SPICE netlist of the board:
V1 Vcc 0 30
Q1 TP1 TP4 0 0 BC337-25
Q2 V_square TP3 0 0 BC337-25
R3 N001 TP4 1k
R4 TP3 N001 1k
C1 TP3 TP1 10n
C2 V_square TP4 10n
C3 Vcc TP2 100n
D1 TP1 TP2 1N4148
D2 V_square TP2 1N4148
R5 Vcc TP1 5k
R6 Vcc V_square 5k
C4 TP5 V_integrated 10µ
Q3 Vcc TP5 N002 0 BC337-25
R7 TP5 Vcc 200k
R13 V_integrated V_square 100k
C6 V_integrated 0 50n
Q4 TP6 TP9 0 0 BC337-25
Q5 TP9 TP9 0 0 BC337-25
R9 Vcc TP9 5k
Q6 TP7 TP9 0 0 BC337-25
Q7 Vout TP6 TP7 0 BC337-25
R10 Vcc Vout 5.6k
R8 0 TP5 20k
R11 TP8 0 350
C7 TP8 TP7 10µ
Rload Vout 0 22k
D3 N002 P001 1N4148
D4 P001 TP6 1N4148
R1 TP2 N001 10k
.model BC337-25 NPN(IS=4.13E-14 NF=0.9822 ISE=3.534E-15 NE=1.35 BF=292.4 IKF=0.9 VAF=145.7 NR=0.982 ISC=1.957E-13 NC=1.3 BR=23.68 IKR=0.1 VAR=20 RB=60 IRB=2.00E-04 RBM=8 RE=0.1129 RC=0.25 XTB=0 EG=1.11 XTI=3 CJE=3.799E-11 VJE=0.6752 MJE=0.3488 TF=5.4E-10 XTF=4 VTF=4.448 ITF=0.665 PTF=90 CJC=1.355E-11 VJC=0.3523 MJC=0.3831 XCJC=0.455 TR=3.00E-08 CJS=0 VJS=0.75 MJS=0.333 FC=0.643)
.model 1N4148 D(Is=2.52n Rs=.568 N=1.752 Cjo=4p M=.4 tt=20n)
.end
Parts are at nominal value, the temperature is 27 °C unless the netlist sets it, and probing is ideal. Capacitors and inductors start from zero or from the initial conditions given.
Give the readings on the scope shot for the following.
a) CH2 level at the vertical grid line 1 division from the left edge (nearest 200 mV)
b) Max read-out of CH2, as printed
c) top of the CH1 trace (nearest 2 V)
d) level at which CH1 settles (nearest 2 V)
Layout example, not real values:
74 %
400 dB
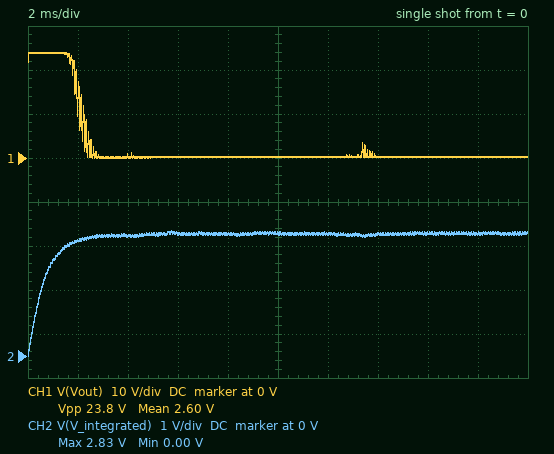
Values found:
2.6 V
2.83 V
24 V
0 V
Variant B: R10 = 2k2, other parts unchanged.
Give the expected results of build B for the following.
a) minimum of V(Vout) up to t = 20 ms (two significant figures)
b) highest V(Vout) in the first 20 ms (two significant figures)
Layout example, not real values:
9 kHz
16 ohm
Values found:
15 V
27 V
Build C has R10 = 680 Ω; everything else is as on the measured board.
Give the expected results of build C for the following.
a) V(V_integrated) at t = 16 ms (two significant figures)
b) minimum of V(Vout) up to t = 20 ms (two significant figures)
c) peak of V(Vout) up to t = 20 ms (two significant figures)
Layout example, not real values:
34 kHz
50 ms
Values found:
2.8 V
25 V
29 V
